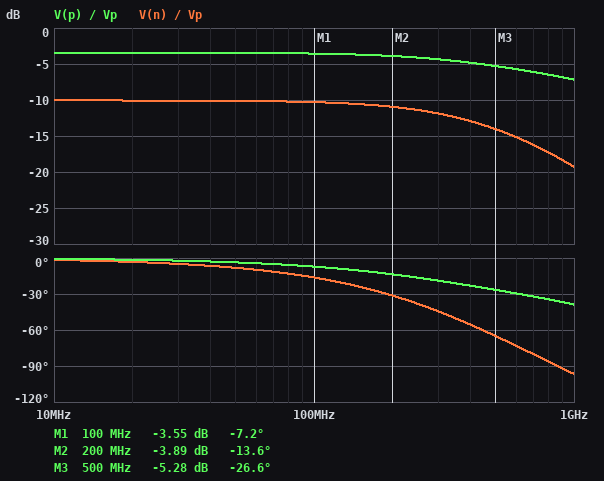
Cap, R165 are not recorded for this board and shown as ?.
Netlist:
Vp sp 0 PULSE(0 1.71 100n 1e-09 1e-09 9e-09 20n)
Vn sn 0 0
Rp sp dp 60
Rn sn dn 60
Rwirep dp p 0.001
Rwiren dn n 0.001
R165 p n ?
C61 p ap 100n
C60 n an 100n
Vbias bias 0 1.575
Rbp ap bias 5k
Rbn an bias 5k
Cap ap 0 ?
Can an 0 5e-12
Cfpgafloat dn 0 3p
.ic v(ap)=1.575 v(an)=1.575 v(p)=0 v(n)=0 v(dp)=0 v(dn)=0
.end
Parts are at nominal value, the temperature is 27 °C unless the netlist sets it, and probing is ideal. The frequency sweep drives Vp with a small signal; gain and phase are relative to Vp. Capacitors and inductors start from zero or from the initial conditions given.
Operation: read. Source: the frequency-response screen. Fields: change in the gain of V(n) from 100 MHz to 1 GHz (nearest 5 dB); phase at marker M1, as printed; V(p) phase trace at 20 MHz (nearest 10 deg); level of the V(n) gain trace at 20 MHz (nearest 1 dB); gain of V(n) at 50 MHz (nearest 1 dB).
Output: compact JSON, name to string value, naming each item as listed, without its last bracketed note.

{"change in the gain of V(n) from 100 MHz to 1 GHz": "-10 dB", "phase at marker M1, as printed": "-7.2 deg", "V(p) phase trace at 20 MHz": "0 deg", "level of the V(n) gain trace at 20 MHz": "-10 dB", "gain of V(n) at 50 MHz": "-10 dB"}
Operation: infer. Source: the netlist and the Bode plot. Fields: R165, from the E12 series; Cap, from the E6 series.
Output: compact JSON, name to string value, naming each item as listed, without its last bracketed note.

{"R165, from the E12 series": "68 Ω", "Cap, from the E6 series": "3.3 pF"}
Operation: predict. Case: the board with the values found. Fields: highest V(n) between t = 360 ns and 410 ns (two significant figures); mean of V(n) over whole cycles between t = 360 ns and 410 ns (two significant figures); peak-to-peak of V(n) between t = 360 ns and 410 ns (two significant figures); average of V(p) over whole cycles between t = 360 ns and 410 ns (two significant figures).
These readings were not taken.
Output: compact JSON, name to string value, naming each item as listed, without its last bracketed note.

{"highest V(n) between t = 360 ns and 410 ns": "540 mV", "mean of V(n) over whole cycles between t = 360 ns and 410 ns": "270 mV", "peak-to-peak of V(n) between t = 360 ns and 410 ns": "540 mV", "average of V(p) over whole cycles between t = 360 ns and 410 ns": "580 mV"}
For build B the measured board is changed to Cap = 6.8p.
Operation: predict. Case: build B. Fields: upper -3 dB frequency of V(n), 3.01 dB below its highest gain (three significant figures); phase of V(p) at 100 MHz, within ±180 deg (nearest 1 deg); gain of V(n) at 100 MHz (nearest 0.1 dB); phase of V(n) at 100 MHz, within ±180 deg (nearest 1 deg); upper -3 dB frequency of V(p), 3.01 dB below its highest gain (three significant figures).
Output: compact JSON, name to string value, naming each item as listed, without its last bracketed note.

{"upper -3 dB frequency of V(n), 3.01 dB below its highest gain": "325 MHz", "phase of V(p) at 100 MHz, within ±180 deg": "-12 deg", "gain of V(n) at 100 MHz": "-10.4 dB", "phase of V(n) at 100 MHz, within ±180 deg": "-21 deg", "upper -3 dB frequency of V(p), 3.01 dB below its highest gain": "444 MHz"}
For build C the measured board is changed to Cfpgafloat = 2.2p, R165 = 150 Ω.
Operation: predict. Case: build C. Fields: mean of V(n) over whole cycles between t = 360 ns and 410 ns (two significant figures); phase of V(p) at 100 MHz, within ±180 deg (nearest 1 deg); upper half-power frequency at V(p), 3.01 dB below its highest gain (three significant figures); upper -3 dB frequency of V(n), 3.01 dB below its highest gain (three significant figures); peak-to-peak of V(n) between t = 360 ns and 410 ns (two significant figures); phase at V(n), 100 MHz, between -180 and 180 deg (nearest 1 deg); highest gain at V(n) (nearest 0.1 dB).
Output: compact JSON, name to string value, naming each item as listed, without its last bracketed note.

{"mean of V(n) over whole cycles between t = 360 ns and 410 ns": "190 mV", "phase of V(p) at 100 MHz, within ±180 deg": "-6 deg", "upper half-power frequency at V(p), 3.01 dB below its highest gain": "931 MHz", "upper -3 dB frequency of V(n), 3.01 dB below its highest gain": "403 MHz", "peak-to-peak of V(n) between t = 360 ns and 410 ns": "370 mV", "phase at V(n), 100 MHz, between -180 and 180 deg": "-17 deg", "highest gain at V(n)": "-13.2 dB"}
